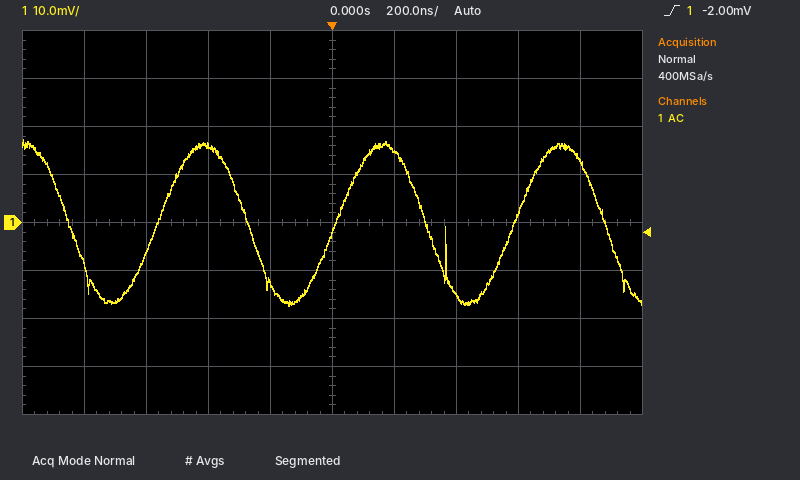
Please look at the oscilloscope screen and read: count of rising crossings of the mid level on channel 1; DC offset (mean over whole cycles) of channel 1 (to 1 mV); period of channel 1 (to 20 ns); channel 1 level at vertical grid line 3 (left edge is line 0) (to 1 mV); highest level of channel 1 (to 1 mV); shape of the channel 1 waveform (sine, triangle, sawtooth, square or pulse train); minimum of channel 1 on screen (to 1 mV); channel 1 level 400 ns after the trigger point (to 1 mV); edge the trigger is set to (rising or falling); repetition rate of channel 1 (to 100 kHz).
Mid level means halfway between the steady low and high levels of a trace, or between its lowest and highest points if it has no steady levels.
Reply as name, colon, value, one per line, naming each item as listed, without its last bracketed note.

count of rising crossings of the mid level on channel 1: 3
DC offset (mean over whole cycles) of channel 1: 0 mV
period of channel 1: 580 ns
channel 1 level at vertical grid line 3 (left edge is line 0): 16 mV
highest level of channel 1: 17 mV
shape of the channel 1 waveform: sine
minimum of channel 1 on screen: -17 mV
channel 1 level 400 ns after the trigger point: -15 mV
edge the trigger is set to: rising
repetition rate of channel 1: 1.7 MHz
